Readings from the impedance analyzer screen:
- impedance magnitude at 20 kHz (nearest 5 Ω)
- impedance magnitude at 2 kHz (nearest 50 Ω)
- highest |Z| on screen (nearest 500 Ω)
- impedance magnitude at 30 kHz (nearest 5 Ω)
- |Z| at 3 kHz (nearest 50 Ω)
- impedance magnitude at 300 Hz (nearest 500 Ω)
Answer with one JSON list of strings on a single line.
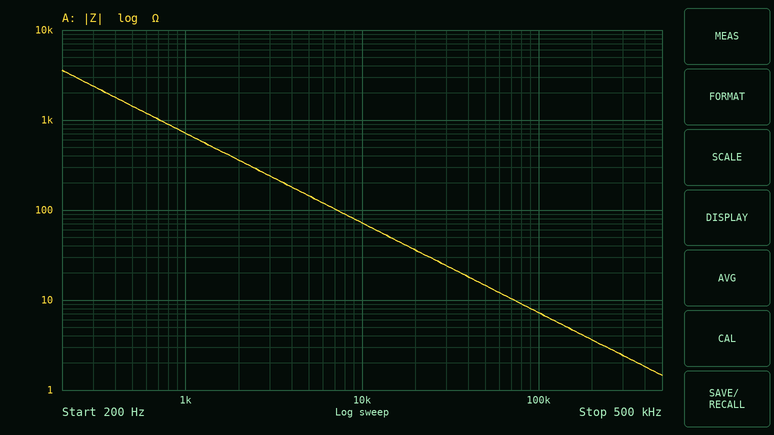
["35 Ω", "350 Ω", "3.5 kΩ", "25 Ω", "250 Ω", "2.5 kΩ"]
